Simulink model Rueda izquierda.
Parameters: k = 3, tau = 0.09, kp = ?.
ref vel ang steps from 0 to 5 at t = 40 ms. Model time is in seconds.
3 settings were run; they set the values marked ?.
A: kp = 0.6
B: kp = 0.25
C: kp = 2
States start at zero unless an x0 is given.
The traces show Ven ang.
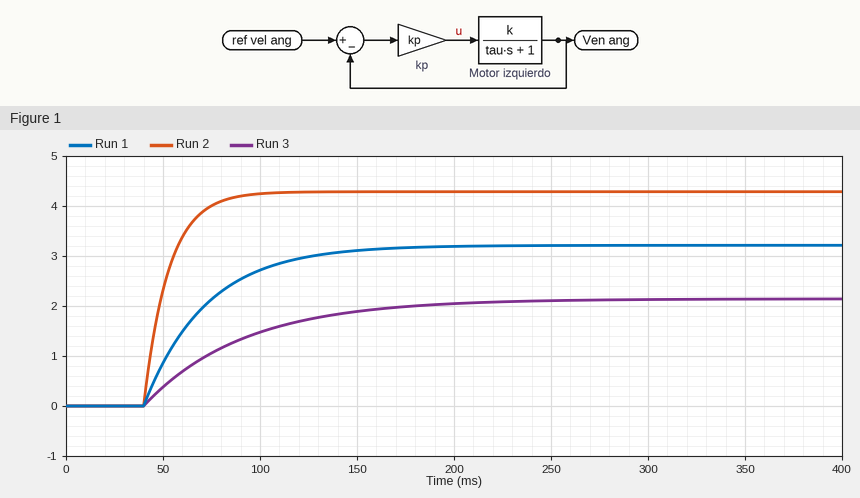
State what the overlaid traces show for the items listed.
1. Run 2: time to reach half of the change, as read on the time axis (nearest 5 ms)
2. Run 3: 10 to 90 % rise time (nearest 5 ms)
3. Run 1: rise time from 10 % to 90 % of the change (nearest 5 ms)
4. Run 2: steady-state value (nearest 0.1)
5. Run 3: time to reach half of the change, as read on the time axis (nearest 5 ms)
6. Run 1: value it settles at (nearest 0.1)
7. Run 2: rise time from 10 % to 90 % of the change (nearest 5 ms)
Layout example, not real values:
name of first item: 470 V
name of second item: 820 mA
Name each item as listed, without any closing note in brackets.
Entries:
Run 2: time to reach half of the change, as read on the time axis: 50 ms
Run 3: 10 to 90 % rise time: 115 ms
Run 1: rise time from 10 % to 90 % of the change: 70 ms
Run 2: steady-state value: 4.3
Run 3: time to reach half of the change, as read on the time axis: 75 ms
Run 1: value it settles at: 3.2
Run 2: rise time from 10 % to 90 % of the change: 30 ms
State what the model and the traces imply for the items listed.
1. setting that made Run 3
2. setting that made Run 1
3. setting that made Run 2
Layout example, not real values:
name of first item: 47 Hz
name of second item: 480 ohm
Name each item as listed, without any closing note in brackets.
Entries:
setting that made Run 3: B
setting that made Run 1: A
setting that made Run 2: C
